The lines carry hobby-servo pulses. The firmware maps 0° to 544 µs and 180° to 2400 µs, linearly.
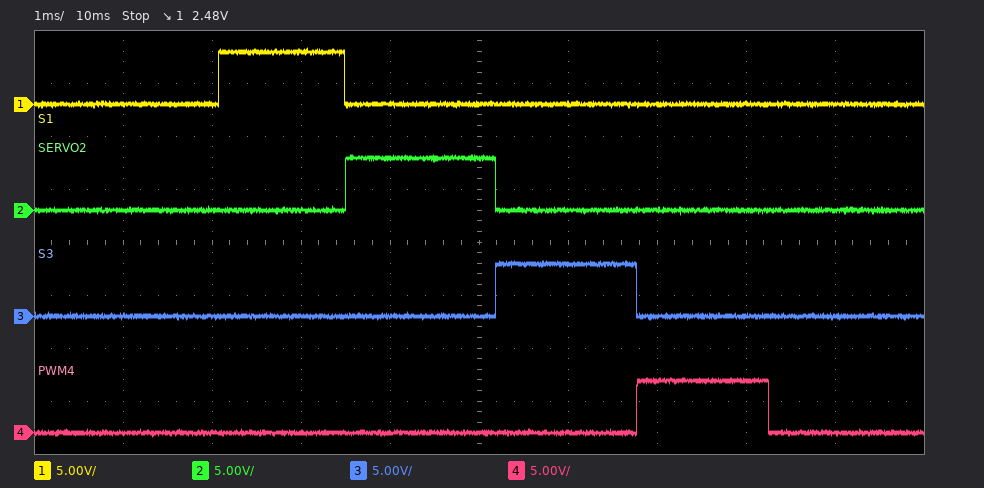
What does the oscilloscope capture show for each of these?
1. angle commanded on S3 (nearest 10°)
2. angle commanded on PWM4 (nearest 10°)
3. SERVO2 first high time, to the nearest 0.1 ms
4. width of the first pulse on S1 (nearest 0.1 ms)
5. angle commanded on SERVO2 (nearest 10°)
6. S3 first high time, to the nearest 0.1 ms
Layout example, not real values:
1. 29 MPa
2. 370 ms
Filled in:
1. 100°
2. 90°
3. 1.7 ms
4. 1.4 ms
5. 110°
6. 1.6 ms
